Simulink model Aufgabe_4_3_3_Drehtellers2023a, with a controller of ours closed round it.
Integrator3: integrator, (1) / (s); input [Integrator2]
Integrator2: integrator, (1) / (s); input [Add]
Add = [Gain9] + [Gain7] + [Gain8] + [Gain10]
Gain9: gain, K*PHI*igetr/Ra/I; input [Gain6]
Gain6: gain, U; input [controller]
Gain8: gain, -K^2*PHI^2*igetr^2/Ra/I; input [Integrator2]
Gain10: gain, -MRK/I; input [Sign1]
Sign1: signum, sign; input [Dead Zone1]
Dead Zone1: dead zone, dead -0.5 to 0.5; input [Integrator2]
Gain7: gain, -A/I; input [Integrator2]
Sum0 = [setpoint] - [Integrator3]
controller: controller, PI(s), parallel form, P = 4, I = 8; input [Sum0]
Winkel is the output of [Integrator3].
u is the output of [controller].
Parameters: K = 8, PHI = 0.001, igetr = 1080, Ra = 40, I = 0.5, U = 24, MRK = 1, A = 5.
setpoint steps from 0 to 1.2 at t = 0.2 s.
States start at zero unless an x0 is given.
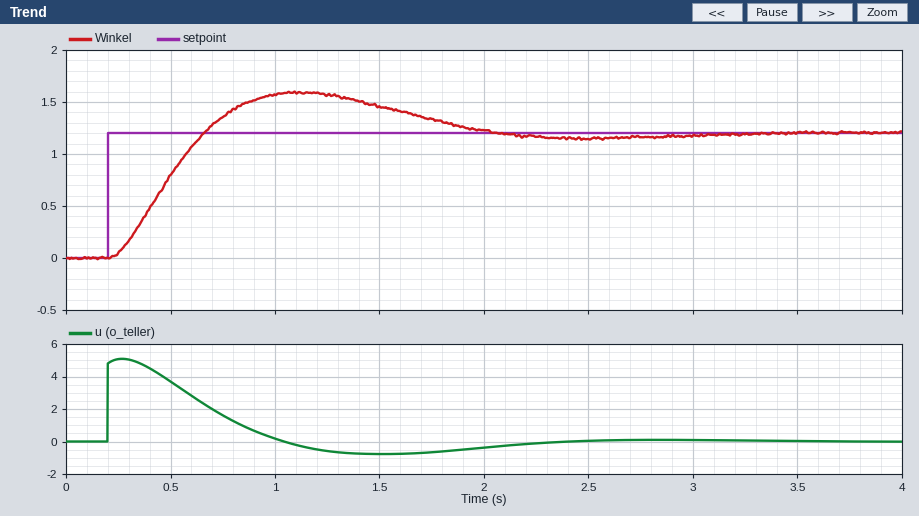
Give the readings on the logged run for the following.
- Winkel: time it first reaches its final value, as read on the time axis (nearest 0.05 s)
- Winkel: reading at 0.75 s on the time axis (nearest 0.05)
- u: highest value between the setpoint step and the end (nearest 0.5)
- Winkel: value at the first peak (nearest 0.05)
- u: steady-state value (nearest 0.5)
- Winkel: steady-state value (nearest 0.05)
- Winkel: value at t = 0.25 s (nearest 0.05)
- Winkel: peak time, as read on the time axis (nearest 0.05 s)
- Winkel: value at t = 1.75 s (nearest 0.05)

0.65 s
1.35
5.0
1.60
0.0
1.20
0.05
1.10 s
1.35
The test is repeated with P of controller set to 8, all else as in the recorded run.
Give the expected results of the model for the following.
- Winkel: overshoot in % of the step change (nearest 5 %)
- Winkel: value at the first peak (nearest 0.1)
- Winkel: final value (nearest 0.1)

15 %
1.4
1.2
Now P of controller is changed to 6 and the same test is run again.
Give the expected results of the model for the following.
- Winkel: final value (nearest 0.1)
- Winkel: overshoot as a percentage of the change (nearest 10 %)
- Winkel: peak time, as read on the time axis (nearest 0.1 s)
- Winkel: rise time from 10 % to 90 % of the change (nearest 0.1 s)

1.2
20 %
0.9 s
0.3 s
